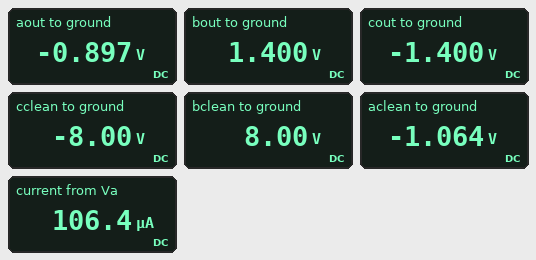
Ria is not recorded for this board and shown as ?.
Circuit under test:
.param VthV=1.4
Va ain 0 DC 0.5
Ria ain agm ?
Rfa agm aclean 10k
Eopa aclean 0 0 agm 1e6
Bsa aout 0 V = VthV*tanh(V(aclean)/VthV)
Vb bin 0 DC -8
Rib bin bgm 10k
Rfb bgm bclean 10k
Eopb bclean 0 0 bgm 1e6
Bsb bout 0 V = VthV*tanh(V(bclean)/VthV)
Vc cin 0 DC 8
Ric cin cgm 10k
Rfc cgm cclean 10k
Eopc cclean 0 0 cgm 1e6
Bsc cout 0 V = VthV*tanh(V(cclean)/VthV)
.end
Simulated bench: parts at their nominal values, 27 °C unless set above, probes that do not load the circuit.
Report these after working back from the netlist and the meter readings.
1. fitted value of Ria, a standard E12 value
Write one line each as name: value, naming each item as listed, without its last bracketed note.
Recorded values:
fitted value of Ria, a standard E12 value: 4.7 kΩ
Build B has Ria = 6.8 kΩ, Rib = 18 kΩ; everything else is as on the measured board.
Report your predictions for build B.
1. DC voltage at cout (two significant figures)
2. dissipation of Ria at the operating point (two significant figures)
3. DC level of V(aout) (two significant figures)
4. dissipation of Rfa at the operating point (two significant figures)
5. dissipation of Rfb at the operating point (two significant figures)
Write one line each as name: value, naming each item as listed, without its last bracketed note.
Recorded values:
DC voltage at cout: -1.4 V
dissipation of Ria at the operating point: 37 µW
DC level of V(aout): -670 mV
dissipation of Rfa at the operating point: 54 µW
dissipation of Rfb at the operating point: 2.0 mW
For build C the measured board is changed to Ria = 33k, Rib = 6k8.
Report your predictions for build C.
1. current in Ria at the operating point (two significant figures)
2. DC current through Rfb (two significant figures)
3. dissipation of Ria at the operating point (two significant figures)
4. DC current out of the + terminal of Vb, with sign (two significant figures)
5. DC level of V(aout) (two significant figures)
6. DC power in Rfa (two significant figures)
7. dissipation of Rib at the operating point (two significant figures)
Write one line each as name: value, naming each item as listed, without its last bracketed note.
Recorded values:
current in Ria at the operating point: 15 µA
DC current through Rfb: 1.2 mA
dissipation of Ria at the operating point: 7.6 µW
DC current out of the + terminal of Vb, with sign: -1.2 mA
DC level of V(aout): -150 mV
DC power in Rfa: 2.3 µW
dissipation of Rib at the operating point: 9.4 mW
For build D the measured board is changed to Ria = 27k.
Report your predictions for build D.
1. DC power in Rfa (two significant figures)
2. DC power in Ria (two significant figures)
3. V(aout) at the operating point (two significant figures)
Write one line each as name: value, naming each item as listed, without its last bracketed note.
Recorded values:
DC power in Rfa: 3.4 µW
DC power in Ria: 9.3 µW
V(aout) at the operating point: -180 mV
